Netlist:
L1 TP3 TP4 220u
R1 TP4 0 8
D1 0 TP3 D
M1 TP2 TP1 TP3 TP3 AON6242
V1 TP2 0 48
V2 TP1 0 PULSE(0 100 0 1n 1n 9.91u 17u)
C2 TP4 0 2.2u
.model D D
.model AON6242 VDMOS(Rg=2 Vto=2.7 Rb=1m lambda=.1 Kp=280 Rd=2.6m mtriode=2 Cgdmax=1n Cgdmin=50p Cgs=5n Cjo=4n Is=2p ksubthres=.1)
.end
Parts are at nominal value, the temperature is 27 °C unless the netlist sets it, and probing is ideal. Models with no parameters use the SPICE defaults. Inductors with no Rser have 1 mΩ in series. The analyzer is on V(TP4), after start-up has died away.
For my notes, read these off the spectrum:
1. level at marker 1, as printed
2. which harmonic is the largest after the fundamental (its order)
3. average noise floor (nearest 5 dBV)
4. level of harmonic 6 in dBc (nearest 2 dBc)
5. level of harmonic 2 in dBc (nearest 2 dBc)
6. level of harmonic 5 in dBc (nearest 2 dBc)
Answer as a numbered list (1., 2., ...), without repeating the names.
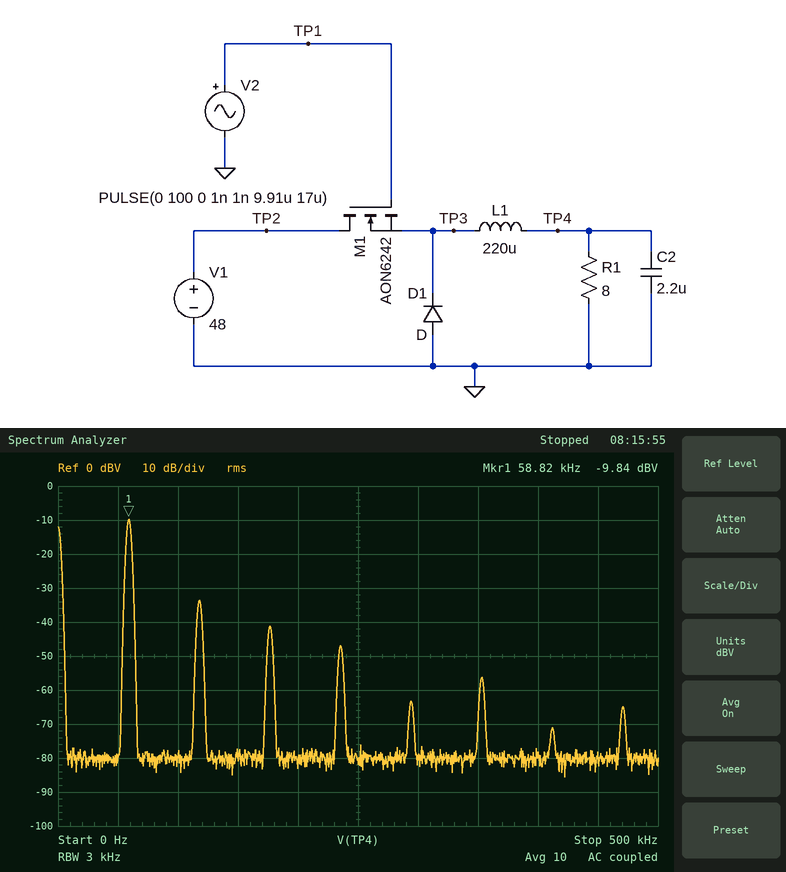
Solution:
1. -9.84 dBV
2. 2
3. -80 dBV
4. -46 dBc
5. -24 dBc
6. -54 dBc
